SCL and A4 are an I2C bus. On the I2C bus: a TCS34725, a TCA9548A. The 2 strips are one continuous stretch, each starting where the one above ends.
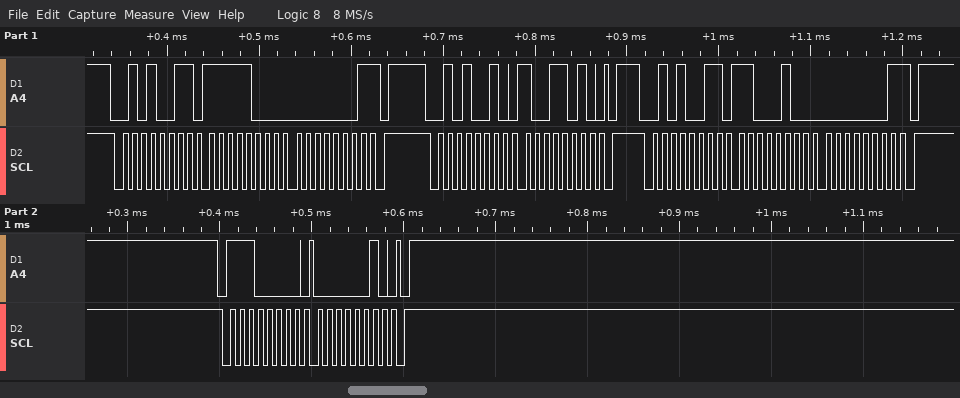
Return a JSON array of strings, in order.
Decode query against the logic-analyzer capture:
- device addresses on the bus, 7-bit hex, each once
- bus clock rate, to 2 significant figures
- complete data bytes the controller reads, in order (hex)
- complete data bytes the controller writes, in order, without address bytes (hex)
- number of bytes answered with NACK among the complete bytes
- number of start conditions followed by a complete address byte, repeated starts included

["0x29 0x70", "100 kHz", "F8 01 C4 01", "9A 02", "2", "4"]
